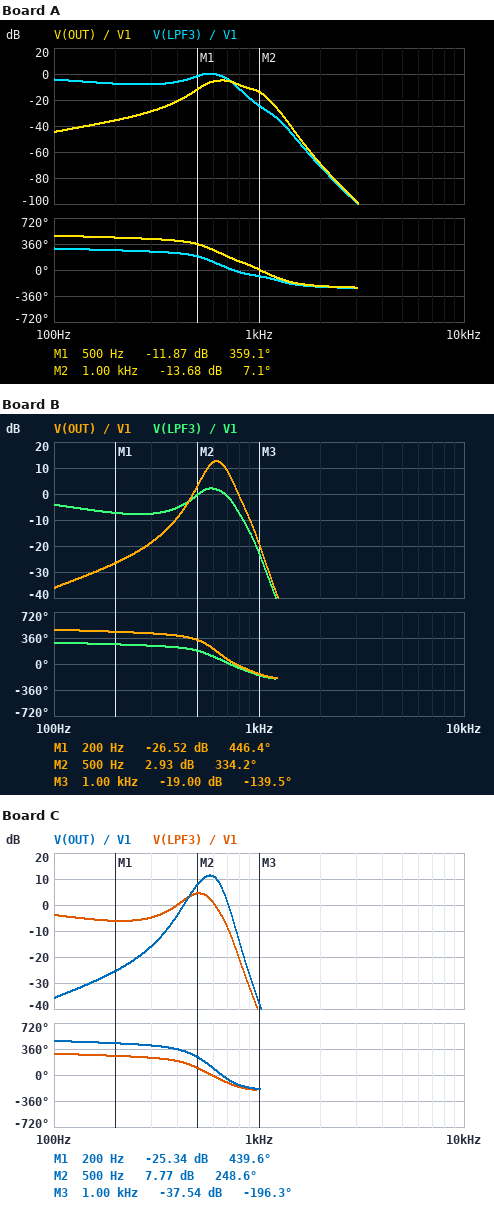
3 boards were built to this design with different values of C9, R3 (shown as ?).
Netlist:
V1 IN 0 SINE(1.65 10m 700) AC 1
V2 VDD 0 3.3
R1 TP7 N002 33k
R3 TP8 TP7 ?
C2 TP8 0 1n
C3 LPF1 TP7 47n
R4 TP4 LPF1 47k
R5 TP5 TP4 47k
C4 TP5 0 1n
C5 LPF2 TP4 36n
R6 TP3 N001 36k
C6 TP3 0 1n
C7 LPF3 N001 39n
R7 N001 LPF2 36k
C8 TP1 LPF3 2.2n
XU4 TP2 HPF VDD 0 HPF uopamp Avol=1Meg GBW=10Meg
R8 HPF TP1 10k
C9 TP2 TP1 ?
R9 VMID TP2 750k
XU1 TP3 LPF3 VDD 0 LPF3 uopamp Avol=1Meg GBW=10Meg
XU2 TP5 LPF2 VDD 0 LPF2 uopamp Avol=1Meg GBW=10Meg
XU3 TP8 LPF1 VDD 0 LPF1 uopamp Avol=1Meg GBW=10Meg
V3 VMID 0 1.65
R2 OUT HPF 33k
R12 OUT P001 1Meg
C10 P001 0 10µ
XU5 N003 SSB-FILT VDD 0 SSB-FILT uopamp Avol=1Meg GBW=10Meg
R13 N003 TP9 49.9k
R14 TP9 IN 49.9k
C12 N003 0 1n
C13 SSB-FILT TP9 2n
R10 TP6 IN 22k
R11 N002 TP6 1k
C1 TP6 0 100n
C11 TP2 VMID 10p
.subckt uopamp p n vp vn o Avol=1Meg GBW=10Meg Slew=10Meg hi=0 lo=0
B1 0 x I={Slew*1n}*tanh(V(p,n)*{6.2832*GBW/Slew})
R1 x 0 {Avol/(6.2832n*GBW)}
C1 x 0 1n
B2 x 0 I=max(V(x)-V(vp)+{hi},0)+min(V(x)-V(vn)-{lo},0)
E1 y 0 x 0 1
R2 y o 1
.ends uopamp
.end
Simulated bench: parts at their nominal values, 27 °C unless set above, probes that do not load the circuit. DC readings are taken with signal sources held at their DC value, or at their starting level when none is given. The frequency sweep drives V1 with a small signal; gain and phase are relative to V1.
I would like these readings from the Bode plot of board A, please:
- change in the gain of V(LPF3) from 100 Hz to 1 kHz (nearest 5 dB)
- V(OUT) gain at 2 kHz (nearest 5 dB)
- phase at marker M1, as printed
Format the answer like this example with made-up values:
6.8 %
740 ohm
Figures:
-20 dB
-70 dB
359.1 deg
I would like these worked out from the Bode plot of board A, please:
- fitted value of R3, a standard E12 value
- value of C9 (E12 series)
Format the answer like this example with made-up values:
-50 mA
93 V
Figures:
10 kΩ
1.5 nF
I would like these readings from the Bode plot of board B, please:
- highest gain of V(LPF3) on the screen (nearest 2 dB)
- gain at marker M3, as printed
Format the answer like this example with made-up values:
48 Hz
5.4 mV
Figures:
2 dB
-19.00 dB
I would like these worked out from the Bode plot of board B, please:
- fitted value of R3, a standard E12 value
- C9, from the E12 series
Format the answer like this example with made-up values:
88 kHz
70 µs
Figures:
18 kΩ
3.9 nF
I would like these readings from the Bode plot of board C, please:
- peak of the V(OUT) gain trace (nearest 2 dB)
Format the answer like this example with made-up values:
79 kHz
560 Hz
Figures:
12 dB
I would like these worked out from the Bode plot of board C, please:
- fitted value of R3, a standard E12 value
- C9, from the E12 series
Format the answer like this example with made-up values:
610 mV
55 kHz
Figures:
68 kΩ
3.9 nF
